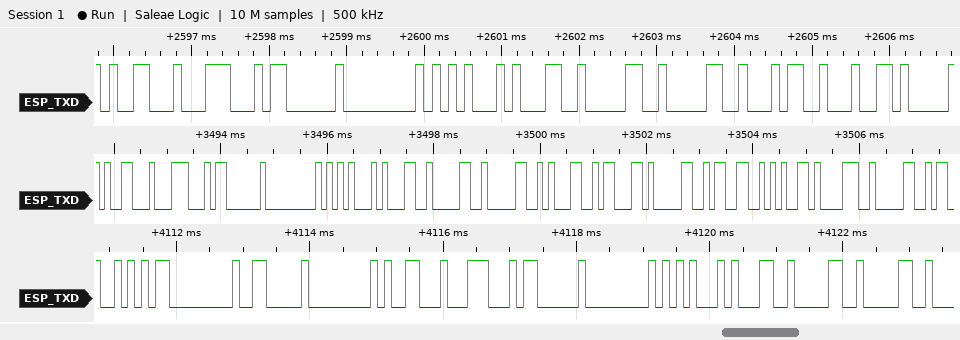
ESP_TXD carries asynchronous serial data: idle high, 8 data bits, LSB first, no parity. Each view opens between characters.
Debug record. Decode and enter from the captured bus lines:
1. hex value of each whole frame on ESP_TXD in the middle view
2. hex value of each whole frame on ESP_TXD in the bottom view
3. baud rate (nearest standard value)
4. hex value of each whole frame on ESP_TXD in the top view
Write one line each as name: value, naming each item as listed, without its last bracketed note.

hex value of each whole frame on ESP_TXD in the middle view: 19, 1C, 03, 00, 15, 31, 30, 30, 31, 63, 30, 33, 65, 38, 30
hex value of each whole frame on ESP_TXD in the bottom view: AA, 00, 06, 00, 19, 1C, 03, 00, 15, 31, 30, 30
baud rate: 9600 baud
hex value of each whole frame on ESP_TXD in the top view: 19, 1C, 03, 00, 15, 31, 30, 30, 34, 64
